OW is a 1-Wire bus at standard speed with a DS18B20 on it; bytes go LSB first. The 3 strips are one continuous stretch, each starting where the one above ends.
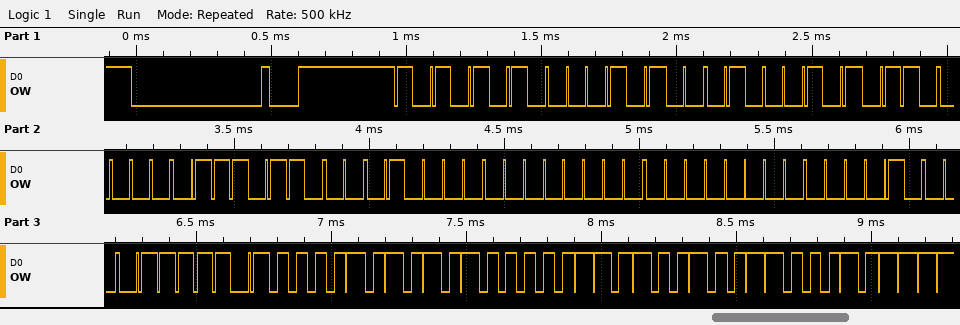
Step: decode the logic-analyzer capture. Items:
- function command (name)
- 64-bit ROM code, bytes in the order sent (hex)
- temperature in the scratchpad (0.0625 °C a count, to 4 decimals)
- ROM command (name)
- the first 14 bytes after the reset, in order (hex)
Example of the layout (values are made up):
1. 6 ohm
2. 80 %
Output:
1. Read Scratchpad
2. 28 A2 06 6E 08 00 00 10
3. 85.0000 °C
4. Match ROM
5. 55 28 A2 06 6E 08 00 00 10 BE 50 05 4B 46
